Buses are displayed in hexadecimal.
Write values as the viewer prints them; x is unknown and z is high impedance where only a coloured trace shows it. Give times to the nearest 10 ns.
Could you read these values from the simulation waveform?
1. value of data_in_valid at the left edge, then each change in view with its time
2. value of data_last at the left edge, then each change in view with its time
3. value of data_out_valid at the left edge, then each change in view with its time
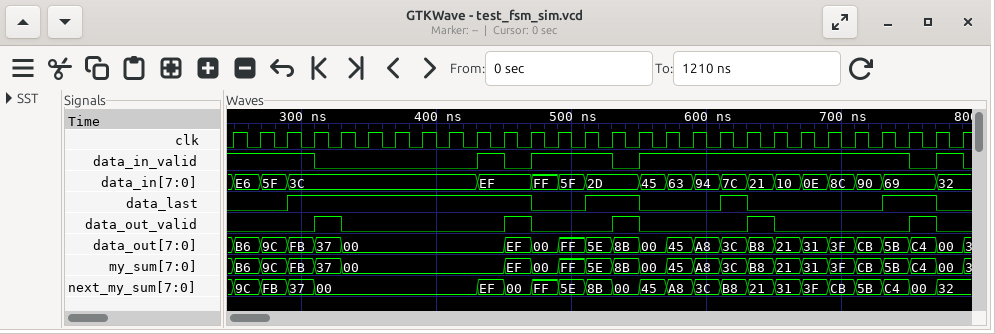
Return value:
1, 0 at 310 ns, 1 at 430 ns, 0 at 450 ns, 1 at 470 ns, 0 at 530 ns, 1 at 550 ns, 0 at 750 ns, 1 at 770 ns, 0 at 790 ns
0, 1 at 290 ns, 0 at 470 ns, 1 at 510 ns, 0 at 550 ns, 1 at 610 ns, 0 at 630 ns, 1 at 730 ns, 0 at 770 ns
0, 1 at 310 ns, 0 at 330 ns, 1 at 450 ns, 0 at 470 ns, 1 at 530 ns, 0 at 550 ns, 1 at 630 ns, 0 at 650 ns, 1 at 750 ns, 0 at 770 ns
